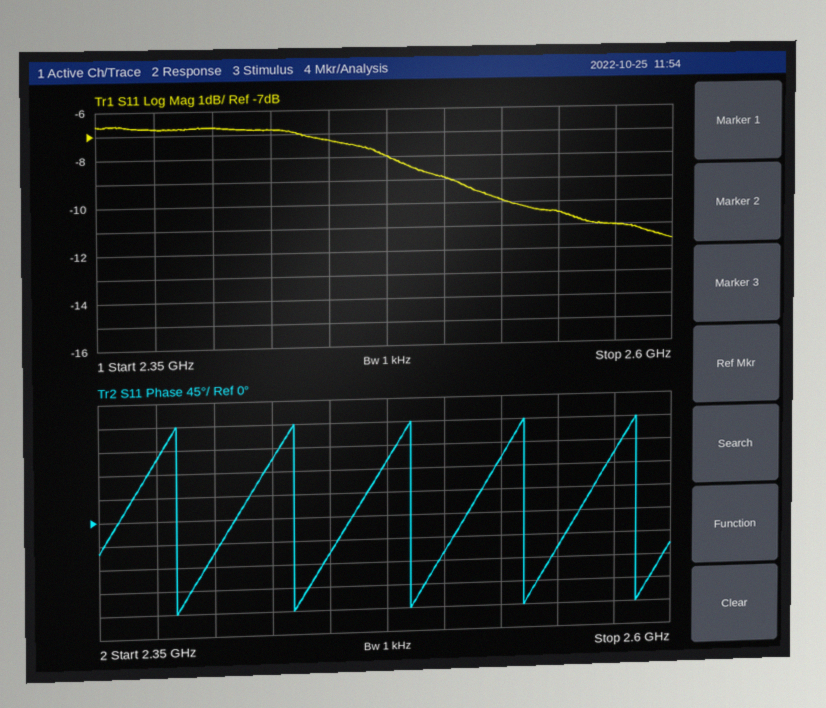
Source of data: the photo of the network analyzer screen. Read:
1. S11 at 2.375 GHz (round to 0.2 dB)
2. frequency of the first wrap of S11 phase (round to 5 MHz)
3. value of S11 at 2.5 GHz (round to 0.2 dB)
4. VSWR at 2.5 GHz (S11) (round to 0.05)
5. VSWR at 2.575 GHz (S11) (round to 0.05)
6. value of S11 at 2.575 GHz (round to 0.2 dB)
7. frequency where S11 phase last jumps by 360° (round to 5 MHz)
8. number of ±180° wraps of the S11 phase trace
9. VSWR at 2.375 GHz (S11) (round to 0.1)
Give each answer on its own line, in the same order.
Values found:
-6.8 dB
2.385 GHz
-9.0 dB
2.10
1.80
-11.0 dB
2.585 GHz
5
2.7
